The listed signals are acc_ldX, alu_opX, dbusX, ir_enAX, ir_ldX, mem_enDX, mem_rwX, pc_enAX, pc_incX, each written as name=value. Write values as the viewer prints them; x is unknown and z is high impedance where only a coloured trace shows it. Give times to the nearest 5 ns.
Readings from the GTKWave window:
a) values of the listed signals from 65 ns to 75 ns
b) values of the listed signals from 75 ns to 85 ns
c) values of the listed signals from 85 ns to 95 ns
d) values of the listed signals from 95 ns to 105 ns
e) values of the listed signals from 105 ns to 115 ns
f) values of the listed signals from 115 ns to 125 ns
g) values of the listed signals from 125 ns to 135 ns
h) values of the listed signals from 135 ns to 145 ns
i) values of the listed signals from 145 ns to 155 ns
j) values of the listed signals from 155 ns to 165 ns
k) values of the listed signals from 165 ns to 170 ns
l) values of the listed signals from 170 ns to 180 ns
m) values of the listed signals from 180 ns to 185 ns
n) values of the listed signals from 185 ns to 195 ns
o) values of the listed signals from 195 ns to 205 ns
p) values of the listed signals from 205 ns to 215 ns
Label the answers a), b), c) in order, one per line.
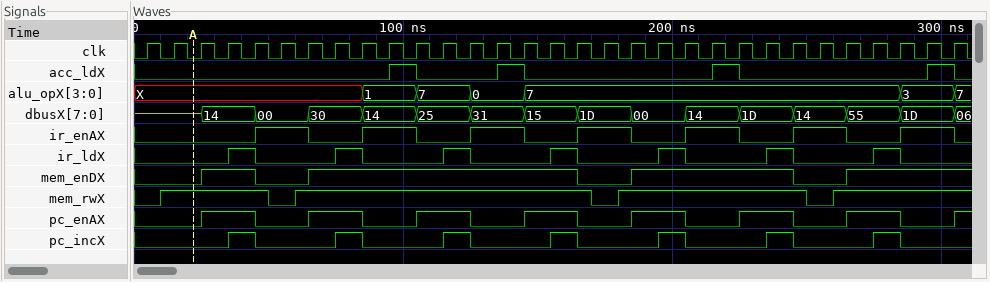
a) acc_ldX=0, alu_opX=X, dbusX=30, ir_enAX=0, ir_ldX=0, mem_enDX=1, mem_rwX=1, pc_enAX=1, pc_incX=0
b) acc_ldX=0, alu_opX=X, dbusX=30, ir_enAX=0, ir_ldX=1, mem_enDX=1, mem_rwX=1, pc_enAX=1, pc_incX=1
c) acc_ldX=0, alu_opX=1, dbusX=14, ir_enAX=1, ir_ldX=0, mem_enDX=1, mem_rwX=1, pc_enAX=0, pc_incX=0
d) acc_ldX=1, alu_opX=1, dbusX=14, ir_enAX=1, ir_ldX=0, mem_enDX=1, mem_rwX=1, pc_enAX=0, pc_incX=0
e) acc_ldX=0, alu_opX=7, dbusX=25, ir_enAX=0, ir_ldX=0, mem_enDX=1, mem_rwX=1, pc_enAX=1, pc_incX=0
f) acc_ldX=0, alu_opX=7, dbusX=25, ir_enAX=0, ir_ldX=1, mem_enDX=1, mem_rwX=1, pc_enAX=1, pc_incX=1
g) acc_ldX=0, alu_opX=0, dbusX=31, ir_enAX=1, ir_ldX=0, mem_enDX=1, mem_rwX=1, pc_enAX=0, pc_incX=0
h) acc_ldX=1, alu_opX=0, dbusX=31, ir_enAX=1, ir_ldX=0, mem_enDX=1, mem_rwX=1, pc_enAX=0, pc_incX=0
i) acc_ldX=0, alu_opX=7, dbusX=15, ir_enAX=0, ir_ldX=0, mem_enDX=1, mem_rwX=1, pc_enAX=1, pc_incX=0
j) acc_ldX=0, alu_opX=7, dbusX=15, ir_enAX=0, ir_ldX=1, mem_enDX=1, mem_rwX=1, pc_enAX=1, pc_incX=1
k) acc_ldX=0, alu_opX=7, dbusX=1D, ir_enAX=1, ir_ldX=0, mem_enDX=0, mem_rwX=1, pc_enAX=0, pc_incX=0
l) acc_ldX=0, alu_opX=7, dbusX=1D, ir_enAX=1, ir_ldX=0, mem_enDX=0, mem_rwX=0, pc_enAX=0, pc_incX=0
m) acc_ldX=0, alu_opX=7, dbusX=1D, ir_enAX=1, ir_ldX=0, mem_enDX=0, mem_rwX=1, pc_enAX=0, pc_incX=0
n) acc_ldX=0, alu_opX=7, dbusX=00, ir_enAX=0, ir_ldX=0, mem_enDX=1, mem_rwX=1, pc_enAX=1, pc_incX=0
o) acc_ldX=0, alu_opX=7, dbusX=00, ir_enAX=0, ir_ldX=1, mem_enDX=1, mem_rwX=1, pc_enAX=1, pc_incX=1
p) acc_ldX=0, alu_opX=7, dbusX=14, ir_enAX=1, ir_ldX=0, mem_enDX=1, mem_rwX=1, pc_enAX=0, pc_incX=0
